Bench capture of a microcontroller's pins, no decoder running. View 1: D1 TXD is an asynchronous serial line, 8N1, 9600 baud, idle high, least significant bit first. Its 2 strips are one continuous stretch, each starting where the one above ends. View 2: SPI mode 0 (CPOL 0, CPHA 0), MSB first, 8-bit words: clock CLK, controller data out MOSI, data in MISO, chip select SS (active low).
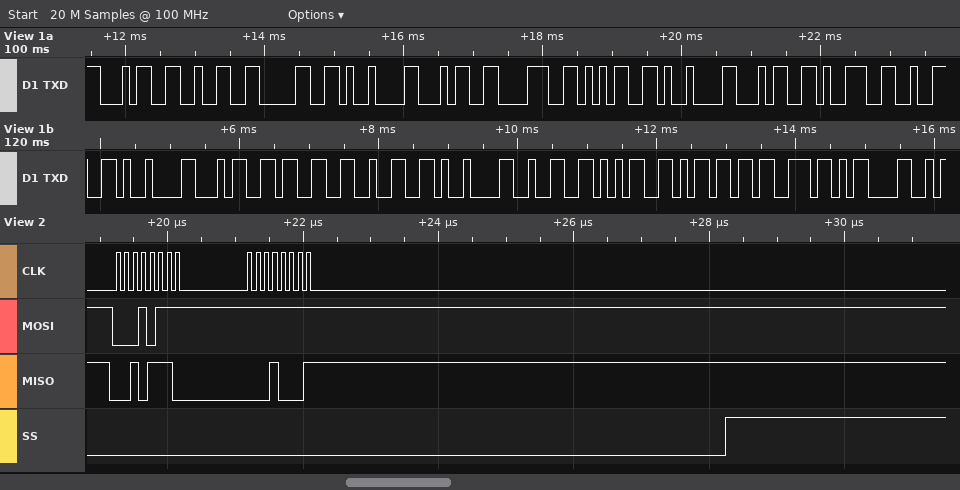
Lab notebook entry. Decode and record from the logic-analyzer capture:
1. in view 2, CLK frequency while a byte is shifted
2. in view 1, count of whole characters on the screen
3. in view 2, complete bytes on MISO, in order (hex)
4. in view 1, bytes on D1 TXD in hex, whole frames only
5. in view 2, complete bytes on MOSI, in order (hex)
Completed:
8 MHz
21
2E 11
34 32 30 09 34 38 35 09 34 39 32 09 34 33 32 09 32 35 6D 73 0D
17 FF
